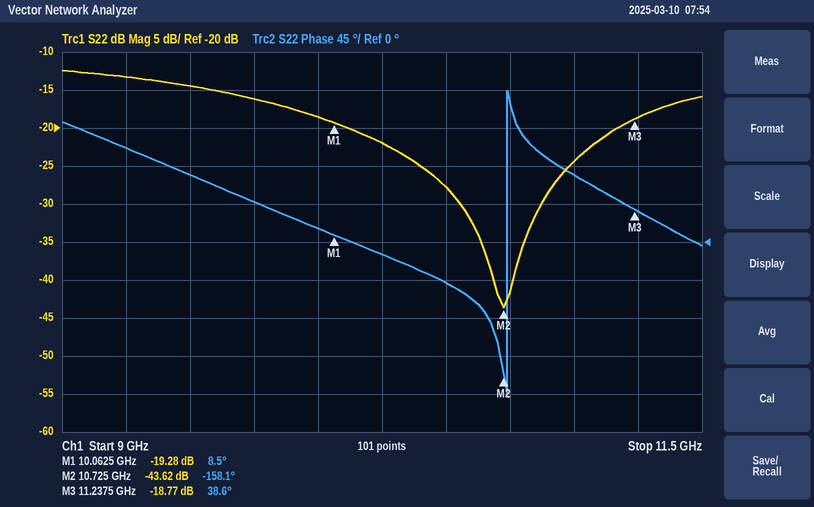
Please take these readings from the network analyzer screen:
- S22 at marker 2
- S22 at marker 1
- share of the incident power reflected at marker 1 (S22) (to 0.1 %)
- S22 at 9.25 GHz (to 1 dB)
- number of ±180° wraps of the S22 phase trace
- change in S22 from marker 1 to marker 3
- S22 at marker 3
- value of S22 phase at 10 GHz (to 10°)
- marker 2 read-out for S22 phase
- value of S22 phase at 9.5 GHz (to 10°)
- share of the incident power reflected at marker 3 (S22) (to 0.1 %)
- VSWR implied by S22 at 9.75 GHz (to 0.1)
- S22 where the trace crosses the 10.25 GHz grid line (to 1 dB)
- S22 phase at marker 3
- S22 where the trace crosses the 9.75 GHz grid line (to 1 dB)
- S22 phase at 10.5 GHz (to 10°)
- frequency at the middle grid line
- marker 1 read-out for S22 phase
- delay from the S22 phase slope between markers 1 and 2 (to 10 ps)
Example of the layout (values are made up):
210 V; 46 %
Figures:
-43.62 dB; -19.28 dB; 1.2 %; -13 dB; 1; 0.51 dB; -18.77 dB; 20°; -158.1°; 80°; 1.3 %; 1.4; -22 dB; 38.6°; -16 dB; -50°; 10.25 GHz; 8.5°; 700 ps
